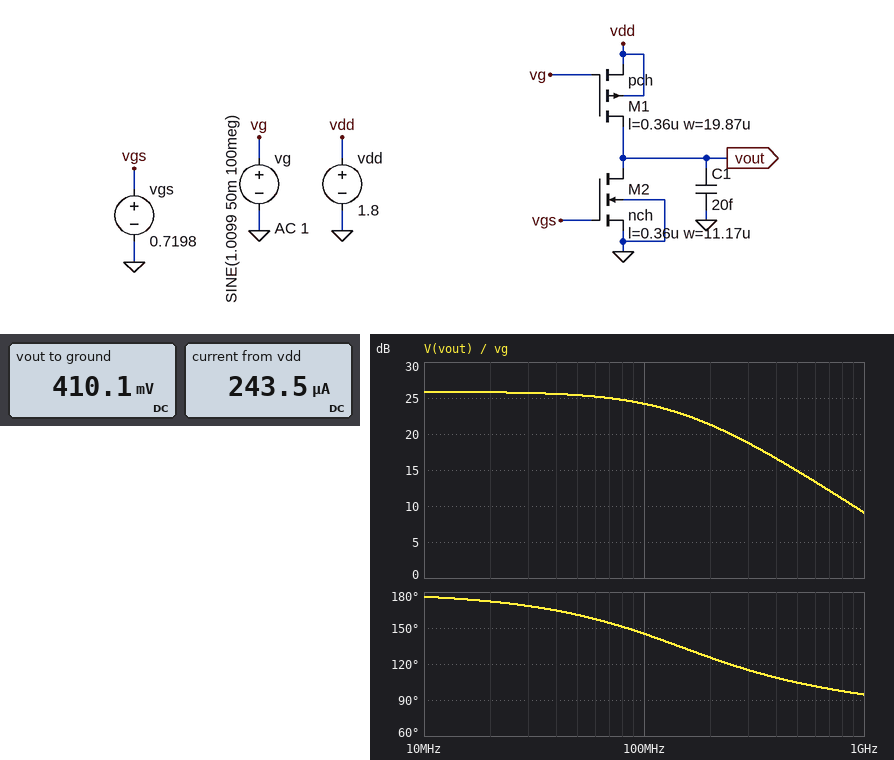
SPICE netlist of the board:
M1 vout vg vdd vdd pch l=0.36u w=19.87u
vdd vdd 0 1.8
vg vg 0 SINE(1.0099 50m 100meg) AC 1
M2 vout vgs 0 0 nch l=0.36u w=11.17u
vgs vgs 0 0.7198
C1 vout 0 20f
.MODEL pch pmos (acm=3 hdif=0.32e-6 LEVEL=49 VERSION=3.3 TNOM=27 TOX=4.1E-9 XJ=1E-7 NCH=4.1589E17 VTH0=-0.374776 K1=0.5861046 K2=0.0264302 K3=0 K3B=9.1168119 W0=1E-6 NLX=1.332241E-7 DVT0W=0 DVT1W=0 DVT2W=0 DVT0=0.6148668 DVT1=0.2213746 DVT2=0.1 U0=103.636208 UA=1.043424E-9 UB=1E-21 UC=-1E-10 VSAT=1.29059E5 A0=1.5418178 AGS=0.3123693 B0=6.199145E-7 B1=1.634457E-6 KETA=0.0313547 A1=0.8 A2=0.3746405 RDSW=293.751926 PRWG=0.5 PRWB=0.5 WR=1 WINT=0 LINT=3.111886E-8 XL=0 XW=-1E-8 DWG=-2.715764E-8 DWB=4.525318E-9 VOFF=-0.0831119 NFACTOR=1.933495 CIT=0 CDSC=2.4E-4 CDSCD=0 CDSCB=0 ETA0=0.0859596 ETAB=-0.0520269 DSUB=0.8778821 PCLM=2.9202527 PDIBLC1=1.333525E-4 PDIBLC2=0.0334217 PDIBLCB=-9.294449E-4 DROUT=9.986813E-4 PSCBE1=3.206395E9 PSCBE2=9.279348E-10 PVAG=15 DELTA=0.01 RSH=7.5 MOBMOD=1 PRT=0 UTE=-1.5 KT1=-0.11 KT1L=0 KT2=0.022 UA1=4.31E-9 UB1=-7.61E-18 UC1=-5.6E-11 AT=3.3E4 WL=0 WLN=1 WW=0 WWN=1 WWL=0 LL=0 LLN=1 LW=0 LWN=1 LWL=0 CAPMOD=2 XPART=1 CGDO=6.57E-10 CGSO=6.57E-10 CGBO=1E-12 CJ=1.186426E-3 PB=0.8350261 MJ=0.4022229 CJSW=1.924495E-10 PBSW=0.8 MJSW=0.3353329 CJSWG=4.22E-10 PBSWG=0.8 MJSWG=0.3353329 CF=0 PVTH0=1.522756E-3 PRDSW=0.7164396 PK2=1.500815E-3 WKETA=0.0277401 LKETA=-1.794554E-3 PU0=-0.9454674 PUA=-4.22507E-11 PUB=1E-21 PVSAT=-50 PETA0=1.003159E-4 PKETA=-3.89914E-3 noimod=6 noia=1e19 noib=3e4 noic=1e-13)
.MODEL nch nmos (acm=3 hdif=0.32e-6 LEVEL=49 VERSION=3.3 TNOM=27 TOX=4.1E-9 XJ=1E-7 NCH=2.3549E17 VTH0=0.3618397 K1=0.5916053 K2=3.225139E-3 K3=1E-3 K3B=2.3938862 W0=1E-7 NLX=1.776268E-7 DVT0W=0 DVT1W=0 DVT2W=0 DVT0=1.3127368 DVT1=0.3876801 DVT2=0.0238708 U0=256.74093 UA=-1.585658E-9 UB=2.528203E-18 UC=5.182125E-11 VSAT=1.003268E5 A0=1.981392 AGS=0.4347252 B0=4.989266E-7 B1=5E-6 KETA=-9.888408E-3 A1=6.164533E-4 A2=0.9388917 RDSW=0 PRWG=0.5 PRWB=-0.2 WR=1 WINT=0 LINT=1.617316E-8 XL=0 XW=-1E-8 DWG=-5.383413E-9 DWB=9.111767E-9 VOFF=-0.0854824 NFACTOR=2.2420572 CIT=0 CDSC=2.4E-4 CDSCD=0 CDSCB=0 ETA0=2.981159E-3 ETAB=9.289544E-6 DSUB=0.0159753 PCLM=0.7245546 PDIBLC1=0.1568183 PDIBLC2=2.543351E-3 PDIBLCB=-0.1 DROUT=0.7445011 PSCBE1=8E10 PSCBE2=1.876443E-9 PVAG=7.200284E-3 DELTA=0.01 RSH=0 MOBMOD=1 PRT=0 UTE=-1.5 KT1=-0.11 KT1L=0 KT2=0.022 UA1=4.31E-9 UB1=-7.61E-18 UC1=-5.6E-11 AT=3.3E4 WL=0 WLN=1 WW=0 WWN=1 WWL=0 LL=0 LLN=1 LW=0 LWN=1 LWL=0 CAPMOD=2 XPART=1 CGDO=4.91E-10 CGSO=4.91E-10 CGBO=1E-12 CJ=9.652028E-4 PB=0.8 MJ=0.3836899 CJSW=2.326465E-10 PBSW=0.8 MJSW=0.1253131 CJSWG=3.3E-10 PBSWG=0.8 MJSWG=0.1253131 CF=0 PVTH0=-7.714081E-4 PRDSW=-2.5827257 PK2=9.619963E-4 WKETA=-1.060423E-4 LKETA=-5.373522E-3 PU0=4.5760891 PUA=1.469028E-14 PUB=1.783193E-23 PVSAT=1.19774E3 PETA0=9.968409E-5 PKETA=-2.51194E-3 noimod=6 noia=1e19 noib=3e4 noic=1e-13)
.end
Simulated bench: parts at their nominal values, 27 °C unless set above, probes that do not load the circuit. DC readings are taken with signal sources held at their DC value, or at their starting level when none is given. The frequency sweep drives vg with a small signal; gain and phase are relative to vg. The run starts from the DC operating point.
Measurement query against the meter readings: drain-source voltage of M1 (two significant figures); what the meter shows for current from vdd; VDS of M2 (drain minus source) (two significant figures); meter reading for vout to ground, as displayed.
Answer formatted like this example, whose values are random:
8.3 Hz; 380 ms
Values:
-1.4 V; 243.5 µA; 410 mV; 410.1 mV
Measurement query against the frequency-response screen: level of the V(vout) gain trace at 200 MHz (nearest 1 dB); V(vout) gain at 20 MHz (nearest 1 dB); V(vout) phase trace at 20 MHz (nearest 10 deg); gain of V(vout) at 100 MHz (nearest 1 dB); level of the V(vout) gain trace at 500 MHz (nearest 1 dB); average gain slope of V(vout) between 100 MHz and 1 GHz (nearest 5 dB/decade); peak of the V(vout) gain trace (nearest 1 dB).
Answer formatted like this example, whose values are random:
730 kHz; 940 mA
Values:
21 dB; 26 dB; 170 deg; 24 dB; 15 dB; -15 dB/decade; 26 dB
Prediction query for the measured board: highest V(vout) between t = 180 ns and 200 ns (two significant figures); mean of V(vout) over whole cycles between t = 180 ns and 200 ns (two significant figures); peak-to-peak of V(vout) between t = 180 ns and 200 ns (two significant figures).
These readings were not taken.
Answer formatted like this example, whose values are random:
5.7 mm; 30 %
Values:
1.3 V; 620 mV; 1.2 V
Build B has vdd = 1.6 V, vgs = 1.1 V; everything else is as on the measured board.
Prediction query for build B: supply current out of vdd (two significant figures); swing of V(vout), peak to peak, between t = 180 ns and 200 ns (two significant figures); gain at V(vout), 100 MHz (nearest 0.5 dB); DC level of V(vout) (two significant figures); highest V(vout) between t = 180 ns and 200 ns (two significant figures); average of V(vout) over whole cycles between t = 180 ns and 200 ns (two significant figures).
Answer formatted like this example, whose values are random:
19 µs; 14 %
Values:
50 µA; 11 mV; -19.5 dB; 8.4 mV; 15 mV; 8.9 mV
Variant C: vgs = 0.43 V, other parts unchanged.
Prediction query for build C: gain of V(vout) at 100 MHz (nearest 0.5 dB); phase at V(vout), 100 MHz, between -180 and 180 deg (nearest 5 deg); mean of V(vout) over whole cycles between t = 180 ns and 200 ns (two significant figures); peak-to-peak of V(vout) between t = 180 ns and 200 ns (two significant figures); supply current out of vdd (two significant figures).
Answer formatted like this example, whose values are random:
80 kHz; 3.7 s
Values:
-34.5 dB; 110 deg; 1.8 V; 1.9 mV; 3.6 µA
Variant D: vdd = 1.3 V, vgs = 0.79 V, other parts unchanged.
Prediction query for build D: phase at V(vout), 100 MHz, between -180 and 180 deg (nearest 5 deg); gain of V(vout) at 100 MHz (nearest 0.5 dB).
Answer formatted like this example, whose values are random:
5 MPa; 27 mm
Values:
105 deg; -51.0 dB
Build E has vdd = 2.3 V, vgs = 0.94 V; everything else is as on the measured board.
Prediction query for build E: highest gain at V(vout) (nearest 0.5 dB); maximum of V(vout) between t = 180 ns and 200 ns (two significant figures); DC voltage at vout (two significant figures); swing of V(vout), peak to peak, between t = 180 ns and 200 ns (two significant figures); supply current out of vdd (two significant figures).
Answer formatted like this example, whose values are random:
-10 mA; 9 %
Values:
-1.5 dB; 2.0 V; 1.9 V; 88 mV; 840 µA
